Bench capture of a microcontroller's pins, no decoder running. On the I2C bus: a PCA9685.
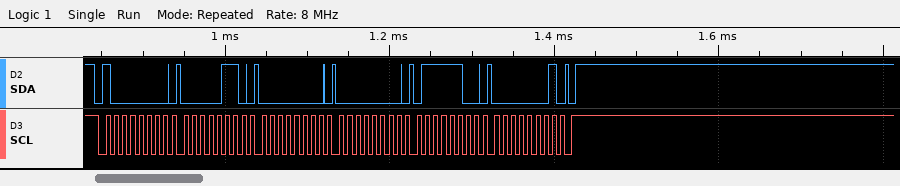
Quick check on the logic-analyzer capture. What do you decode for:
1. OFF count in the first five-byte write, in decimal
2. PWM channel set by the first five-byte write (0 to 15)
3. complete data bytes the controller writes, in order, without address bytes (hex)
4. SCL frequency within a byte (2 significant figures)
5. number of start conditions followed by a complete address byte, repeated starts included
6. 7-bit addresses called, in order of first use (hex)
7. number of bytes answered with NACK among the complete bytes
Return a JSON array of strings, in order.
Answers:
["380", "0", "06 00 00 7C 01", "100 kHz", "1", "0x40", "0"]
